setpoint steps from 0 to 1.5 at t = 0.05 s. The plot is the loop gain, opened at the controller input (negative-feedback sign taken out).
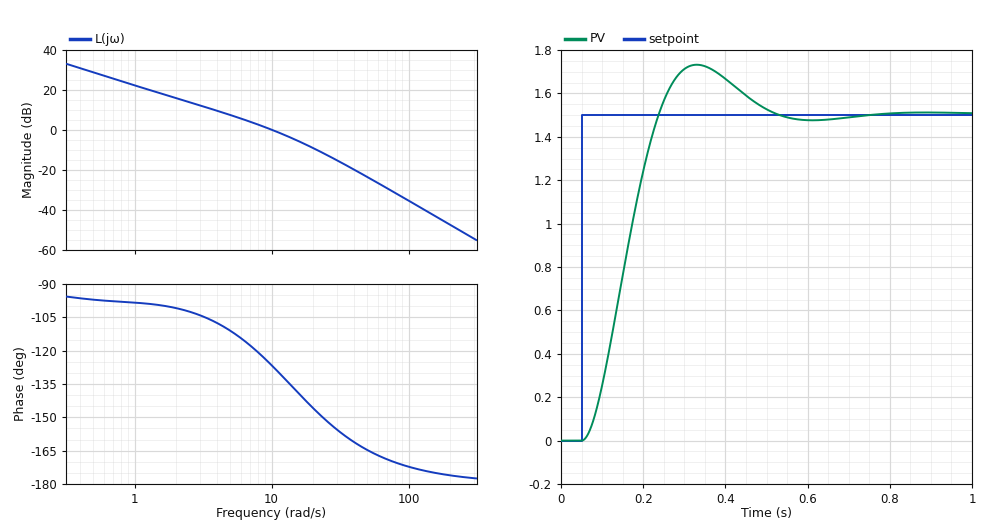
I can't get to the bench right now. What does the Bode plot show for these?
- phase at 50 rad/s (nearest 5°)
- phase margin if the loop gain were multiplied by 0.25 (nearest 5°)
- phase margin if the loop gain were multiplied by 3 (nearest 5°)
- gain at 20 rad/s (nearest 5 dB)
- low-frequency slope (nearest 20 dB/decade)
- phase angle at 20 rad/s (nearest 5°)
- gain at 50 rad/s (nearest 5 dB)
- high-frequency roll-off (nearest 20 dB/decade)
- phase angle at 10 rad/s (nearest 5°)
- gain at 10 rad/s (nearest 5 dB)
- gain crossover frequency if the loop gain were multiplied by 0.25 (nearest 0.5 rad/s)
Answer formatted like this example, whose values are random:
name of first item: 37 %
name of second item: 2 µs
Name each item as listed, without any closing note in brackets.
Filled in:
phase at 50 rad/s: -165°
phase margin if the loop gain were multiplied by 0.25: 75°
phase margin if the loop gain were multiplied by 3: 35°
gain at 20 rad/s: -10 dB
low-frequency slope: -20 dB/decade
phase angle at 20 rad/s: -145°
gain at 50 rad/s: -25 dB
high-frequency roll-off: -40 dB/decade
phase angle at 10 rad/s: -125°
gain at 10 rad/s: 0 dB
gain crossover frequency if the loop gain were multiplied by 0.25: 3.0 rad/s
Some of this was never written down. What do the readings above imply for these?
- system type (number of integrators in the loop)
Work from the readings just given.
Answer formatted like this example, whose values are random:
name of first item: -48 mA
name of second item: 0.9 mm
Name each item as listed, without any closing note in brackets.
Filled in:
system type: 1
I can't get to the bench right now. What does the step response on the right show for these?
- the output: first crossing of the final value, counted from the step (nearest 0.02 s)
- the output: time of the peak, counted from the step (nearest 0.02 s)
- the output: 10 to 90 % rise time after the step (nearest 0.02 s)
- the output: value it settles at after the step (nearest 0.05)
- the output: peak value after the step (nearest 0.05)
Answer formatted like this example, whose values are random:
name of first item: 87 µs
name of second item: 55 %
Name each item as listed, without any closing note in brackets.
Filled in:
the output: first crossing of the final value, counted from the step: 0.18 s
the output: time of the peak, counted from the step: 0.28 s
the output: 10 to 90 % rise time after the step: 0.12 s
the output: value it settles at after the step: 1.50
the output: peak value after the step: 1.75
